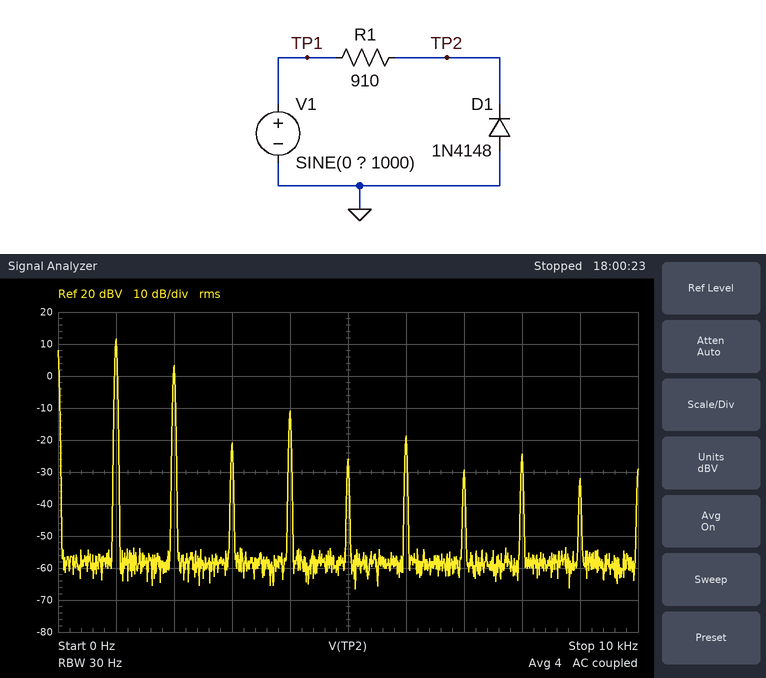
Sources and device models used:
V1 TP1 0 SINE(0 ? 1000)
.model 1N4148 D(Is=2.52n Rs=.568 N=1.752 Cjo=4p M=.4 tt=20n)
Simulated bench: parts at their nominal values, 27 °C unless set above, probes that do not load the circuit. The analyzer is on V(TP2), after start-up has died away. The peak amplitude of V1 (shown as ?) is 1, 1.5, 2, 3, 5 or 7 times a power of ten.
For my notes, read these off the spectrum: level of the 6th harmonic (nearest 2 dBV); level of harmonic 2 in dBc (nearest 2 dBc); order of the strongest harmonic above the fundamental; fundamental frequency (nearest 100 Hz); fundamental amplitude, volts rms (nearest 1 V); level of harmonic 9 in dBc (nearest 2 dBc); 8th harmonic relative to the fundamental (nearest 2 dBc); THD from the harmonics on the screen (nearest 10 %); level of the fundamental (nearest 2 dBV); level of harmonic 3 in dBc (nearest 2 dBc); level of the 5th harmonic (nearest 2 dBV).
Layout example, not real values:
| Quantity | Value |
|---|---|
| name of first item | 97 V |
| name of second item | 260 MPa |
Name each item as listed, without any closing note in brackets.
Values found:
| Quantity | Value |
|---|---|
| level of the 6th harmonic | -18 dBV |
| level of harmonic 2 in dBc | -8 dBc |
| order of the strongest harmonic above the fundamental | 2 |
| fundamental frequency | 1.0 kHz |
| fundamental amplitude, volts rms | 4 V |
| level of harmonic 9 in dBc | -44 dBc |
| 8th harmonic relative to the fundamental | -36 dBc |
| THD from the harmonics on the screen | 40 % |
| level of the fundamental | 12 dBV |
| level of harmonic 3 in dBc | -32 dBc |
| level of the 5th harmonic | -26 dBV |
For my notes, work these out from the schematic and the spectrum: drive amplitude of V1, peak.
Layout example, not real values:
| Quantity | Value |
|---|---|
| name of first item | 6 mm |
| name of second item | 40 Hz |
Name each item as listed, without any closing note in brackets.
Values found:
| Quantity | Value |
|---|---|
| drive amplitude of V1, peak | 10 V |
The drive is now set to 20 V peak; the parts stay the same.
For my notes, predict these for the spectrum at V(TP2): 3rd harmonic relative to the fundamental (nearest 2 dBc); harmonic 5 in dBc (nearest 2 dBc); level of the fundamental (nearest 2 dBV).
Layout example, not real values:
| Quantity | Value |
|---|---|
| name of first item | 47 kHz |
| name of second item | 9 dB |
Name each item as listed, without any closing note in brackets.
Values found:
| Quantity | Value |
|---|---|
| 3rd harmonic relative to the fundamental | -38 dBc |
| harmonic 5 in dBc | -42 dBc |
| level of the fundamental | 18 dBV |
